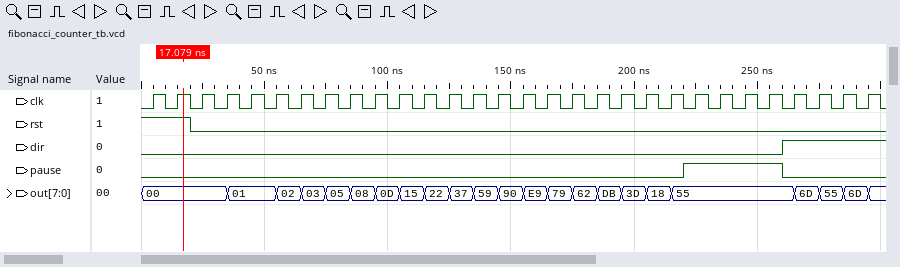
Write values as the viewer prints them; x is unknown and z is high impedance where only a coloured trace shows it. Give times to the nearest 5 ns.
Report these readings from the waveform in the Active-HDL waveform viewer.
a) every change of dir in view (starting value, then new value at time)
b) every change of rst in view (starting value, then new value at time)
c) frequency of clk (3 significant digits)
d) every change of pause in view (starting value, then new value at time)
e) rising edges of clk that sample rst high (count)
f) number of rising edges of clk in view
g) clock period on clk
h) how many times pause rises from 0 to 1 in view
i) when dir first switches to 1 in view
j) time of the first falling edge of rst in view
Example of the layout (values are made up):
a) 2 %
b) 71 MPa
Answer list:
a) 0, 1 at 260 ns
b) 1, 0 at 20 ns
c) 100 MHz
d) 0, 1 at 220 ns, 0 at 260 ns
e) 2
f) 30
g) 10 ns
h) 1
i) 260 ns
j) 20 ns
